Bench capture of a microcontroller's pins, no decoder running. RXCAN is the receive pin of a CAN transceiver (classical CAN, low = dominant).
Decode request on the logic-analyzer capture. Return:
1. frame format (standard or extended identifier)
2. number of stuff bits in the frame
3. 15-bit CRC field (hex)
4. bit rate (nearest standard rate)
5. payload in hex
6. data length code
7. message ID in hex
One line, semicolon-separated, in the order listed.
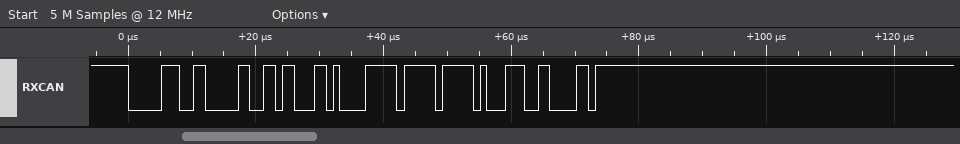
standard; 5; 0x0E61; 1000 kbit/s; D8 D0 FF FF; 4; 0x066
